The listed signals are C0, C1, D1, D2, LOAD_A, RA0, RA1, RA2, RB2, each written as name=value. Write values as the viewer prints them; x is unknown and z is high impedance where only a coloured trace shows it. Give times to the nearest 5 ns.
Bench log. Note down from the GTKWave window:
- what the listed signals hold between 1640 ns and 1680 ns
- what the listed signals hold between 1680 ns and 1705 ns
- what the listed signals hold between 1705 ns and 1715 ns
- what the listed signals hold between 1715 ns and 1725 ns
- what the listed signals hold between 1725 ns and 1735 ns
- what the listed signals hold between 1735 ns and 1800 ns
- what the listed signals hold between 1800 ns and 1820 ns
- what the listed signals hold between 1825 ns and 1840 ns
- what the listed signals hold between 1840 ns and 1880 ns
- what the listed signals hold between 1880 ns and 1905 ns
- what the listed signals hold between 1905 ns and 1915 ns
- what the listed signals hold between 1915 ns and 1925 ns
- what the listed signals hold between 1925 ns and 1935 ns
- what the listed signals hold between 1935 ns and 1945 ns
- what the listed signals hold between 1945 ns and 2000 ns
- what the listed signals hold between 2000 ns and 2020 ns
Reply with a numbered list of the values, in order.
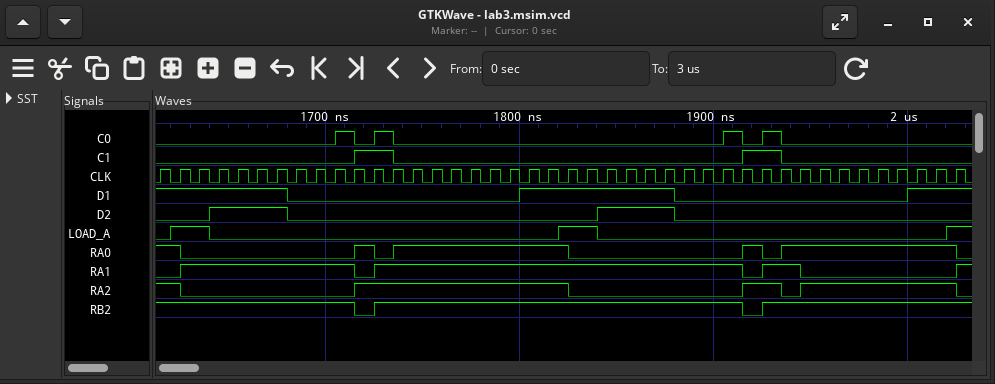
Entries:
1. C0=0, C1=0, D1=1, D2=1, LOAD_A=0, RA0=0, RA1=1, RA2=0, RB2=1
2. C0=0, C1=0, D1=0, D2=0, LOAD_A=0, RA0=0, RA1=1, RA2=0, RB2=1
3. C0=1, C1=0, D1=0, D2=0, LOAD_A=0, RA0=0, RA1=1, RA2=0, RB2=1
4. C0=0, C1=1, D1=0, D2=0, LOAD_A=0, RA0=1, RA1=0, RA2=1, RB2=0
5. C0=1, C1=1, D1=0, D2=0, LOAD_A=0, RA0=0, RA1=1, RA2=1, RB2=1
6. C0=0, C1=0, D1=0, D2=0, LOAD_A=0, RA0=1, RA1=1, RA2=1, RB2=1
7. C0=0, C1=0, D1=1, D2=0, LOAD_A=0, RA0=1, RA1=1, RA2=1, RB2=1
8. C0=0, C1=0, D1=1, D2=0, LOAD_A=1, RA0=0, RA1=1, RA2=0, RB2=1
9. C0=0, C1=0, D1=1, D2=1, LOAD_A=0, RA0=0, RA1=1, RA2=0, RB2=1
10. C0=0, C1=0, D1=0, D2=0, LOAD_A=0, RA0=0, RA1=1, RA2=0, RB2=1
11. C0=1, C1=0, D1=0, D2=0, LOAD_A=0, RA0=0, RA1=1, RA2=0, RB2=1
12. C0=0, C1=1, D1=0, D2=0, LOAD_A=0, RA0=1, RA1=0, RA2=1, RB2=0
13. C0=1, C1=1, D1=0, D2=0, LOAD_A=0, RA0=0, RA1=1, RA2=1, RB2=1
14. C0=0, C1=0, D1=0, D2=0, LOAD_A=0, RA0=1, RA1=1, RA2=0, RB2=1
15. C0=0, C1=0, D1=0, D2=0, LOAD_A=0, RA0=1, RA1=0, RA2=1, RB2=1
16. C0=0, C1=0, D1=1, D2=0, LOAD_A=0, RA0=1, RA1=0, RA2=1, RB2=1
